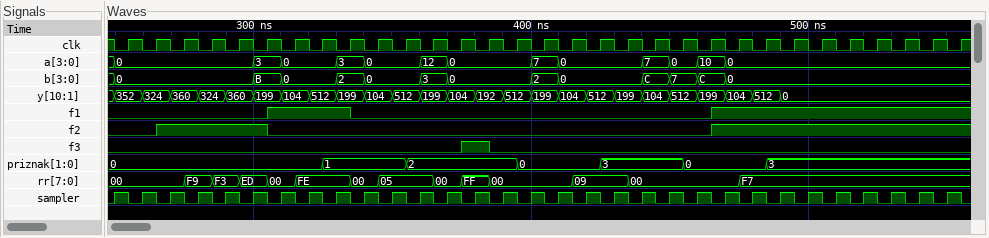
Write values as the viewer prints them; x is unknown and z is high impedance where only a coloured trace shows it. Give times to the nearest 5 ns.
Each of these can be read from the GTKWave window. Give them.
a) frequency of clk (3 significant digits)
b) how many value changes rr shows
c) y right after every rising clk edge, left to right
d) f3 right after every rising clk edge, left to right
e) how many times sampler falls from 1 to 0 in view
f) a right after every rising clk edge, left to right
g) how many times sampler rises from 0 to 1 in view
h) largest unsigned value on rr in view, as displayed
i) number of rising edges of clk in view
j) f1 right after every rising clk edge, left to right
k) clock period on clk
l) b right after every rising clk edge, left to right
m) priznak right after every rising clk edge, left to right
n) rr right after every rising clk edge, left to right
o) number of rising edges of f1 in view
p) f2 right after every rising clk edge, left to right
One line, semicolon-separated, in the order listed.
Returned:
100 MHz; 13; 352, 324, 360, 324, 360, 199, 104, 512, 199, 104, 512, 199, 104, 192, 512, 199, 104, 512, 199, 104, 512, 199, 104, 512, 0, 0, 0, 0, 0, 0, 0; 0 0 0 0 0 0 0 0 0 0 0 0 1 0 0 0 0 0 0 0 0 0 0 0 0 0 0 0 0 0 0; 31; 0, 0, 0, 0, 0, 3, 0, 0, 3, 0, 0, 12, 0, 0, 0, 7, 0, 0, 0, 7, 0, 10, 0, 0, 0, 0, 0, 0, 0, 0, 0; 31; FF; 31; 0 0 0 0 0 1 1 1 0 0 0 0 0 0 0 0 0 0 0 0 0 1 1 1 1 1 1 1 1 1 1; 10 ns; 0, 0, 0, 0, 0, B, 0, 0, 2, 0, 0, 3, 0, 0, 0, 2, 0, 0, 0, C, 7, C, 0, 0, 0, 0, 0, 0, 0, 0, 0; 0, 0, 0, 0, 0, 0, 0, 1, 1, 1, 2, 2, 2, 2, 0, 0, 0, 3, 3, 3, 0, 0, 0, 3, 3, 3, 3, 3, 3, 3, 3; 00, 00, F9, F3, ED, 00, FE, FE, 00, 05, 05, 00, FF, 00, 00, 00, 09, 09, 00, 00, 00, 00, F7, F7, F7, F7, F7, F7, F7, F7, F7; 2; 0 1 1 1 1 0 0 0 0 0 0 0 0 0 0 0 0 0 0 0 0 1 1 1 1 1 1 1 1 1 1
